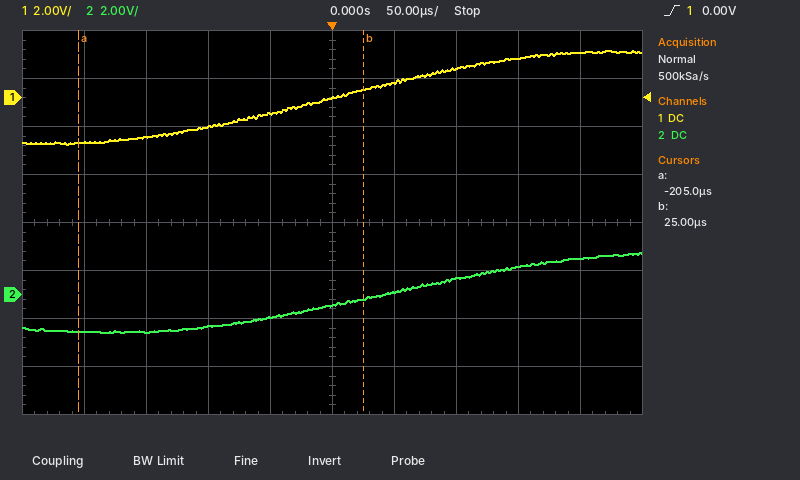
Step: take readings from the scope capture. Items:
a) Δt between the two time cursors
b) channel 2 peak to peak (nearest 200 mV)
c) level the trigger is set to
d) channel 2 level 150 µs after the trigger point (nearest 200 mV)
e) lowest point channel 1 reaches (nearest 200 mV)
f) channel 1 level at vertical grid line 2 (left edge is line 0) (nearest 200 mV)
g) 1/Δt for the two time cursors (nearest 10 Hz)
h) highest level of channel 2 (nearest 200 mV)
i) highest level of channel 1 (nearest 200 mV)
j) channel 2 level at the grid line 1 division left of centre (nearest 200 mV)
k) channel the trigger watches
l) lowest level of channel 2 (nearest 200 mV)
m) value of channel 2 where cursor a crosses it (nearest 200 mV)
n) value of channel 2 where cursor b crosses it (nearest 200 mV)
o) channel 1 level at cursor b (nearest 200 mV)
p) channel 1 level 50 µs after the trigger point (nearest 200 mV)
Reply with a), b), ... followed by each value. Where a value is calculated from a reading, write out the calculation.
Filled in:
a) 25 µs − (-205 µs) = 230 µs
b) 1.8 V − (-1.6 V) = 3.4 V
c) 0.00 V
d) 1.2 V
e) -2.0 V
f) -1.6 V
g) 1 / 230 µs ≈ 4.35 kHz
h) 1.8 V
i) 2.0 V
j) -1.0 V
k) channel 1
l) -1.6 V
m) -1.6 V
n) -200 mV
o) 400 mV
p) 600 mV
